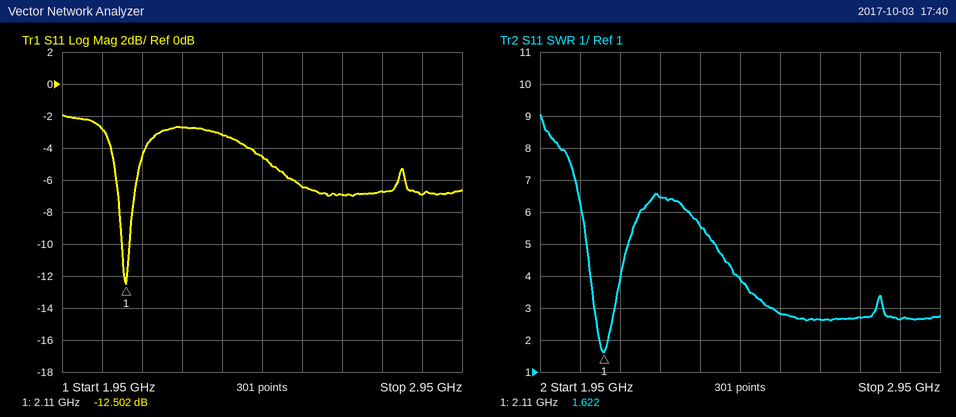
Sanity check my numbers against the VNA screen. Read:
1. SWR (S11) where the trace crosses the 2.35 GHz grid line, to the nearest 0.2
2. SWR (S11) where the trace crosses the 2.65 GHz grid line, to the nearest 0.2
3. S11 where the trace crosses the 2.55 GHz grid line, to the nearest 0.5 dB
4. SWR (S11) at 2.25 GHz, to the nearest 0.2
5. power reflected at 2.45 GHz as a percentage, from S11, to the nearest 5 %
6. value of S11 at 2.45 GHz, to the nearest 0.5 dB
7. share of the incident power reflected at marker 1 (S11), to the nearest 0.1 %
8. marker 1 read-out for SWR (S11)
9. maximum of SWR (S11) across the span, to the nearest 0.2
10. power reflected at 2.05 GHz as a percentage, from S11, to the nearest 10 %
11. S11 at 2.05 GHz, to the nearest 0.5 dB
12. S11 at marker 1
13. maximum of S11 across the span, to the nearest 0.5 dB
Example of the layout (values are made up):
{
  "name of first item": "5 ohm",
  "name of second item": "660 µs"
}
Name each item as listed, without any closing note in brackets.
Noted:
{
  "SWR (S11) where the trace crosses the 2.35 GHz grid line, to the nearest 0.2": "5.6",
  "SWR (S11) where the trace crosses the 2.65 GHz grid line, to the nearest 0.2": "2.6",
  "S11 where the trace crosses the 2.55 GHz grid line, to the nearest 0.5 dB": "-6.5 dB",
  "SWR (S11) at 2.25 GHz, to the nearest 0.2": "6.4",
  "power reflected at 2.45 GHz as a percentage, from S11, to the nearest 5 %": "35 %",
  "value of S11 at 2.45 GHz, to the nearest 0.5 dB": "-4.5 dB",
  "share of the incident power reflected at marker 1 (S11), to the nearest 0.1 %": "5.6 %",
  "marker 1 read-out for SWR": "1.622",
  "maximum of SWR (S11) across the span, to the nearest 0.2": "9.0",
  "power reflected at 2.05 GHz as a percentage, from S11, to the nearest 10 %": "50 %",
  "S11 at 2.05 GHz, to the nearest 0.5 dB": "-3.0 dB",
  "S11 at marker 1": "-12.502 dB",
  "maximum of S11 across the span, to the nearest 0.5 dB": "-2.0 dB"
}
